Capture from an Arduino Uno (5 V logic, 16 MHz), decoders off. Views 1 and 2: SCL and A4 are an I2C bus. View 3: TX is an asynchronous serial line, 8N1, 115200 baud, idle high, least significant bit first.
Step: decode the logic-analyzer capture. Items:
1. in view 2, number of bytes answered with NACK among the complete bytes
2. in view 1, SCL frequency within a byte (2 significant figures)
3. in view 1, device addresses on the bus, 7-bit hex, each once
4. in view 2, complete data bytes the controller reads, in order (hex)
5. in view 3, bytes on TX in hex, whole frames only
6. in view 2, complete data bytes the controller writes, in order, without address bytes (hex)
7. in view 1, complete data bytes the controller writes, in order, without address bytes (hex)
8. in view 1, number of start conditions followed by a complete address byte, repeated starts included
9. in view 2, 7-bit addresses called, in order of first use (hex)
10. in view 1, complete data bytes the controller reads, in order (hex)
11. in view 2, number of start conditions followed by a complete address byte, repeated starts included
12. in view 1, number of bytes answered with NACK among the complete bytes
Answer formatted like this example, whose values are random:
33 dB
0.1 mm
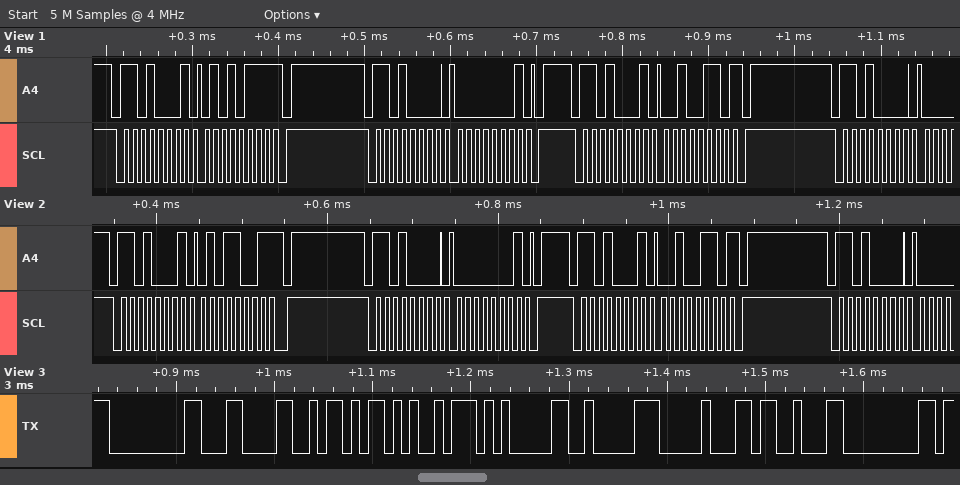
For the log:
2
100 kHz
0x68
59 26
0x00 0x0C 0x5A 0xA5 0x05 0x82 0x10 0x13 0x00
01
01
4
0x68
57 26
4
2
